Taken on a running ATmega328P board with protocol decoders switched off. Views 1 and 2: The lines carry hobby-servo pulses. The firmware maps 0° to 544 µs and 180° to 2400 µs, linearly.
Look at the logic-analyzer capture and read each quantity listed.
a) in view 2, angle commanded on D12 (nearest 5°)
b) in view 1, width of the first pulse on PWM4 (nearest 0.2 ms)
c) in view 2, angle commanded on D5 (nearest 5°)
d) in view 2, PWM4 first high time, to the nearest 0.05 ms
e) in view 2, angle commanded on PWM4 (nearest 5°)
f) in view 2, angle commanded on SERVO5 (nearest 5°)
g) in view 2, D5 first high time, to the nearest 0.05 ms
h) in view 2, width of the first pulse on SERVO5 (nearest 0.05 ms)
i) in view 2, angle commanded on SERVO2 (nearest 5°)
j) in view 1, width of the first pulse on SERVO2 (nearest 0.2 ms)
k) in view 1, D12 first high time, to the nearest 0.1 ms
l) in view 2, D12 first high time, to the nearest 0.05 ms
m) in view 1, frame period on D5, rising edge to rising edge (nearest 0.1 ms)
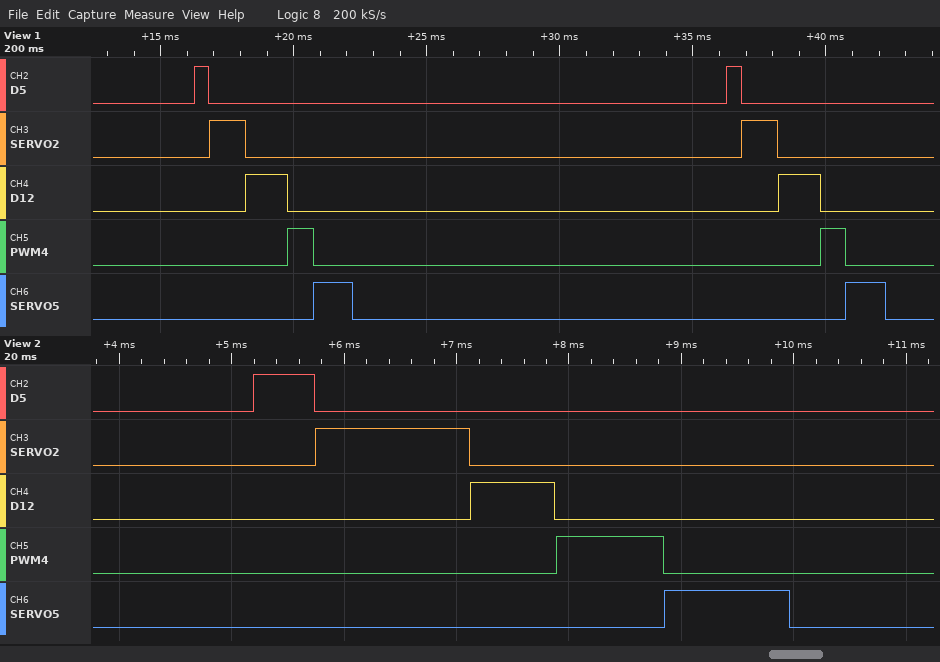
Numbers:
20°
1.0 ms
0°
0.95 ms
40°
55°
0.55 ms
1.10 ms
80°
1.4 ms
1.6 ms
0.75 ms
20.0 ms
